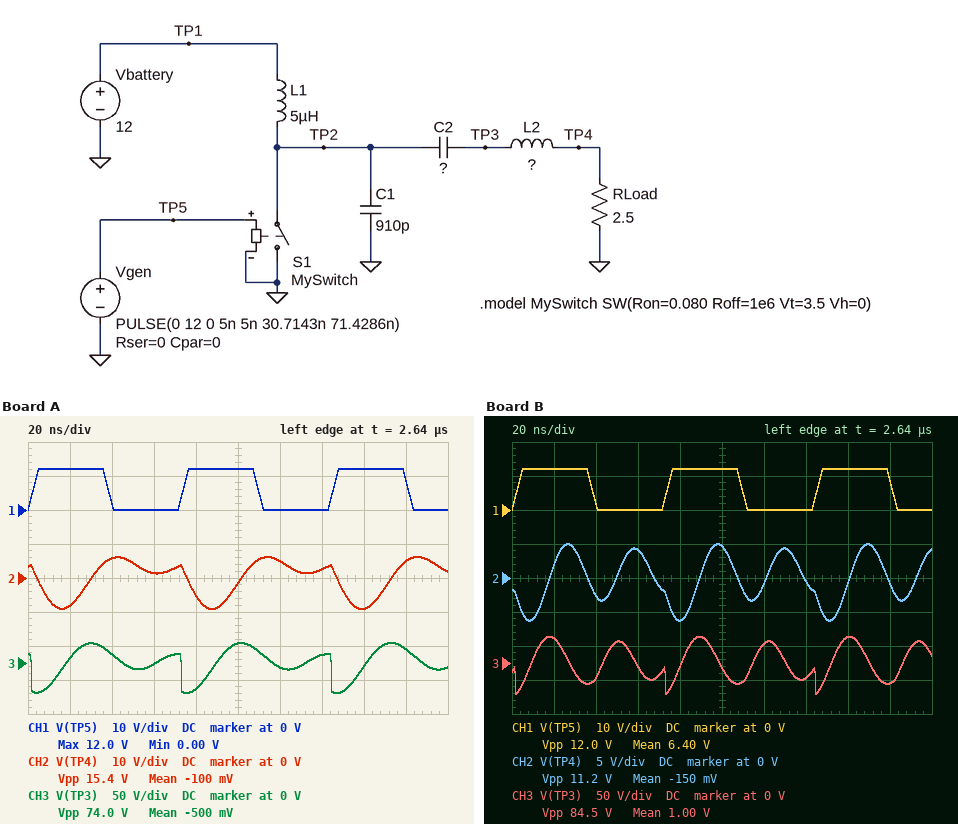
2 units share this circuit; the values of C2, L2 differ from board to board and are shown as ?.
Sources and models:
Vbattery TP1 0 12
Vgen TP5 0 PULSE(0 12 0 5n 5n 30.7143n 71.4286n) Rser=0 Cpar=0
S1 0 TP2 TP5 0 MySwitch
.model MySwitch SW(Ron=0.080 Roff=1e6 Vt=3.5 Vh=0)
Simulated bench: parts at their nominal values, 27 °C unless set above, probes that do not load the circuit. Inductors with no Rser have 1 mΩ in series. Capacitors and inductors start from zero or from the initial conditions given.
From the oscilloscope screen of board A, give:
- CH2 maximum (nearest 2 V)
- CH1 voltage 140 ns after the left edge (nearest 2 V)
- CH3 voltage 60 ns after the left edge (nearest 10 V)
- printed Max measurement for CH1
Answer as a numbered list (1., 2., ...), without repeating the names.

1. 6 V
2. 0 V
3. 0 V
4. 12.0 V
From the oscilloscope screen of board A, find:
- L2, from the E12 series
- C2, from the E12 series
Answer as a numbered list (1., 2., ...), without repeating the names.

1. 82 nH
2. 820 pF
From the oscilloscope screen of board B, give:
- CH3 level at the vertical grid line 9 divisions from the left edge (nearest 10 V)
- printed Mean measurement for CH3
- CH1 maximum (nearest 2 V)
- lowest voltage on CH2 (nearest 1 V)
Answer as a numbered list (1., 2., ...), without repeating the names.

1. -30 V
2. 1.00 V
3. 12 V
4. -6 V
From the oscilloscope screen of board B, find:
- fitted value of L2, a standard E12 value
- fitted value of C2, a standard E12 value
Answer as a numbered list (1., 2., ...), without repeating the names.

1. 100 nH
2. 330 pF
